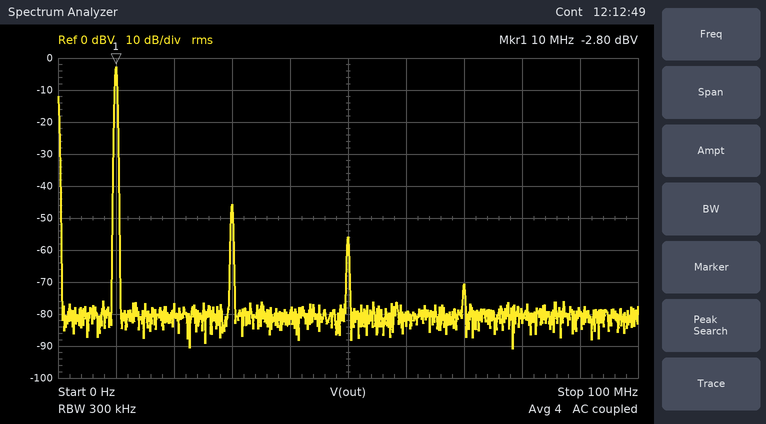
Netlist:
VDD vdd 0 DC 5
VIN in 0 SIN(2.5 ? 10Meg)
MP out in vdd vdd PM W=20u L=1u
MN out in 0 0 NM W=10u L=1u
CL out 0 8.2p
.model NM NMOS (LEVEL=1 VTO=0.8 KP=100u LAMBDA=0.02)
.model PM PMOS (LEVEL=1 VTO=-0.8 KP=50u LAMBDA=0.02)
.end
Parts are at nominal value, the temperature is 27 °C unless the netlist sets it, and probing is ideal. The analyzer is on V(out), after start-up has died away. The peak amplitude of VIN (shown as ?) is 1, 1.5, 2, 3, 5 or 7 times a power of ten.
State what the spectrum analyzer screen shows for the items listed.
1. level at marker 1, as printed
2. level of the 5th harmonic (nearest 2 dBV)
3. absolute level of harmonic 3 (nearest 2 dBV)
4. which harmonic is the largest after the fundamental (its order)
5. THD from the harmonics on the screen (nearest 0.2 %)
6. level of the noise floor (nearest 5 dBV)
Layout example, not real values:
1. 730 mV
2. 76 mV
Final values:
1. -2.80 dBV
2. -56 dBV
3. -46 dBV
4. 3
5. 0.8 %
6. -80 dBV
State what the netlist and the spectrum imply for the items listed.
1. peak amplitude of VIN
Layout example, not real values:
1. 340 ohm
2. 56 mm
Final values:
1. 150 mV
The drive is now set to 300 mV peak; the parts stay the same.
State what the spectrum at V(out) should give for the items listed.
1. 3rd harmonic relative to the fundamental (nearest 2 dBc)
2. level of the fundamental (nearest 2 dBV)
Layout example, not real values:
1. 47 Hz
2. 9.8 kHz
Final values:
1. -24 dBc
2. 2 dBV
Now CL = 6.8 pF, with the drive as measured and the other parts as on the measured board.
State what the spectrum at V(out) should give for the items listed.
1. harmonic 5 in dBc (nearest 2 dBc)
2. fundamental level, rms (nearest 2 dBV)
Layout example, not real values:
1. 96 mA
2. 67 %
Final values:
1. -48 dBc
2. -2 dBV
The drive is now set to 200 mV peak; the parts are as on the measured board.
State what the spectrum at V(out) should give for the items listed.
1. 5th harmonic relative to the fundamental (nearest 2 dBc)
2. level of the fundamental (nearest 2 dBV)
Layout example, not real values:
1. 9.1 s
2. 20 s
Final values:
1. -48 dBc
2. 0 dBV
